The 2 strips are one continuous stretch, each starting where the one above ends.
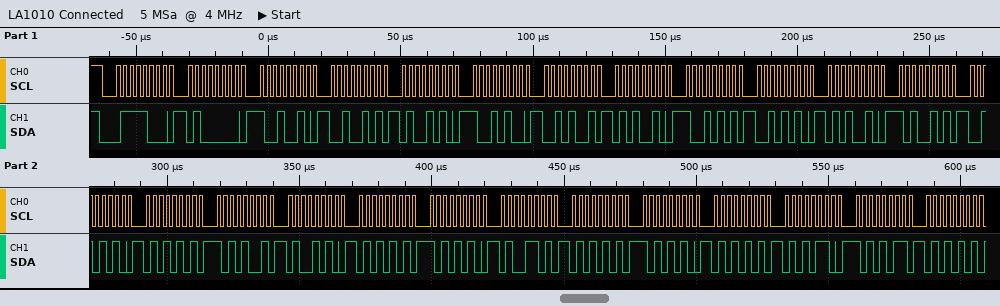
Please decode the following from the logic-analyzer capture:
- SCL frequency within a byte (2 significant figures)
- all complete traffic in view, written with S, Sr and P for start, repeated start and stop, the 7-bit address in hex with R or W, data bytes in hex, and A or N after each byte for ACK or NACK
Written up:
400 kHz
S 3CW A 40 A 92 A 25 A 4A A 94 A 29 A 52 A 95 A 2A A 52 A A5 A 2A A 55 A A9 A 4A A 55 A AA A 4D A 55 A AA A 55 A 56 A AB A 55 A
